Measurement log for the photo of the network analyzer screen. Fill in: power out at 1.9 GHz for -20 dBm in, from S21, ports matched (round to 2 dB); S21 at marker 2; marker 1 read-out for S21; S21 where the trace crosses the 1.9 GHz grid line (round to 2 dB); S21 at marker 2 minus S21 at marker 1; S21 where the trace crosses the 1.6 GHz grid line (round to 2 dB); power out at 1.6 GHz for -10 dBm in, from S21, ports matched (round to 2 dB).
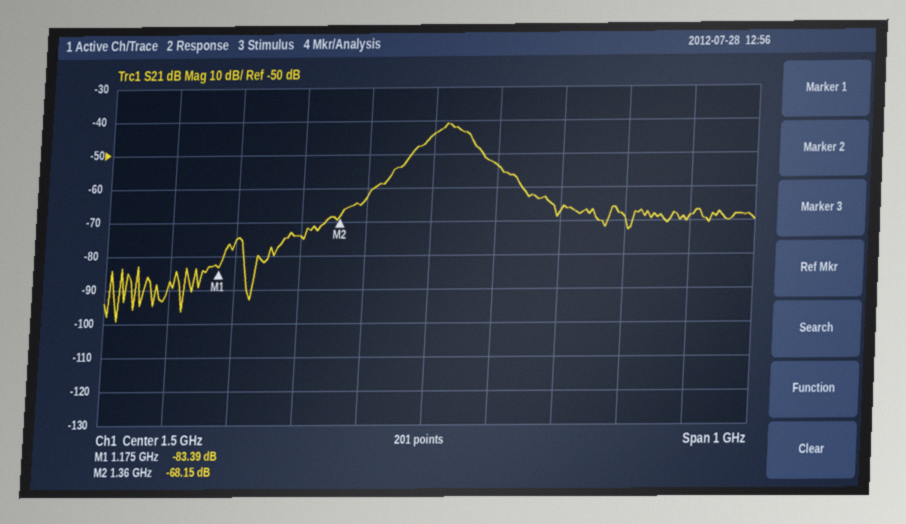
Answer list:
-88 dBm
-68.15 dB
-83.39 dB
-68 dB
15.24 dB
-54 dB
-64 dBm
